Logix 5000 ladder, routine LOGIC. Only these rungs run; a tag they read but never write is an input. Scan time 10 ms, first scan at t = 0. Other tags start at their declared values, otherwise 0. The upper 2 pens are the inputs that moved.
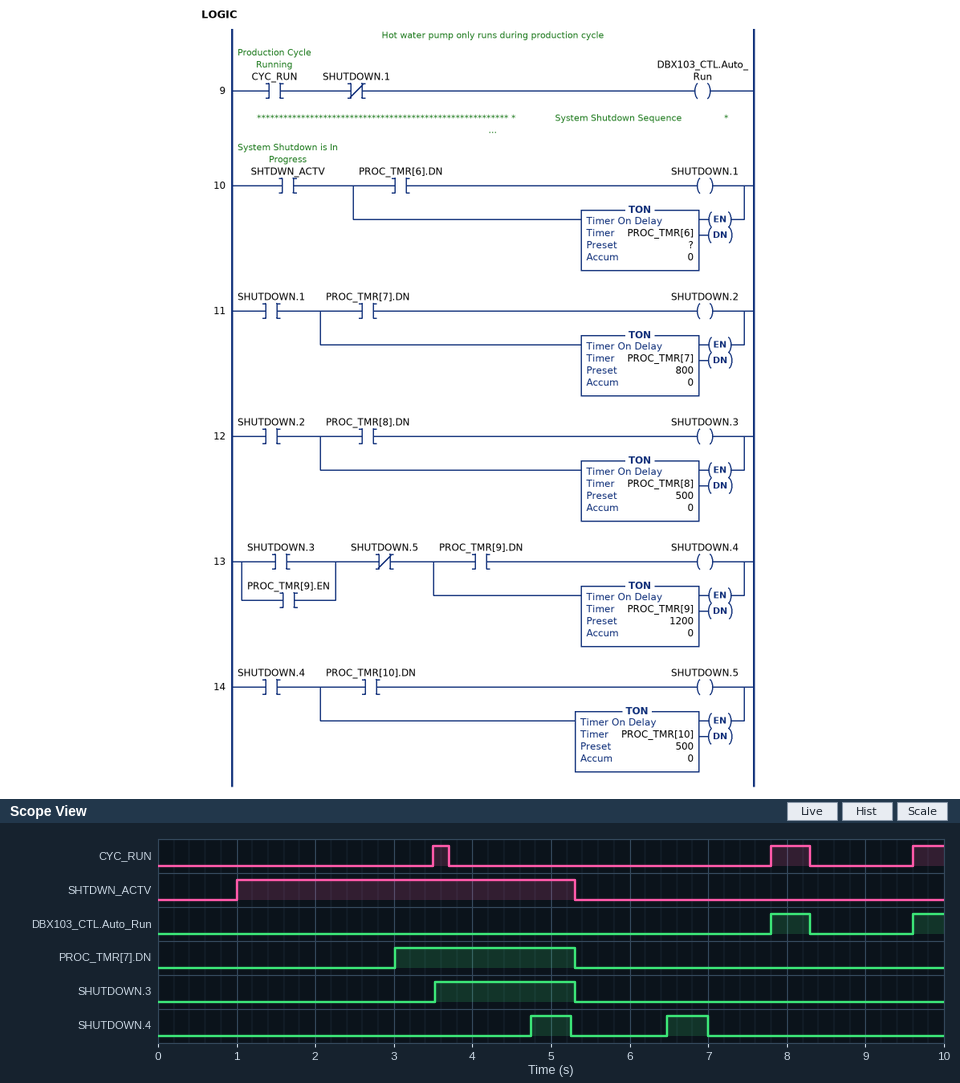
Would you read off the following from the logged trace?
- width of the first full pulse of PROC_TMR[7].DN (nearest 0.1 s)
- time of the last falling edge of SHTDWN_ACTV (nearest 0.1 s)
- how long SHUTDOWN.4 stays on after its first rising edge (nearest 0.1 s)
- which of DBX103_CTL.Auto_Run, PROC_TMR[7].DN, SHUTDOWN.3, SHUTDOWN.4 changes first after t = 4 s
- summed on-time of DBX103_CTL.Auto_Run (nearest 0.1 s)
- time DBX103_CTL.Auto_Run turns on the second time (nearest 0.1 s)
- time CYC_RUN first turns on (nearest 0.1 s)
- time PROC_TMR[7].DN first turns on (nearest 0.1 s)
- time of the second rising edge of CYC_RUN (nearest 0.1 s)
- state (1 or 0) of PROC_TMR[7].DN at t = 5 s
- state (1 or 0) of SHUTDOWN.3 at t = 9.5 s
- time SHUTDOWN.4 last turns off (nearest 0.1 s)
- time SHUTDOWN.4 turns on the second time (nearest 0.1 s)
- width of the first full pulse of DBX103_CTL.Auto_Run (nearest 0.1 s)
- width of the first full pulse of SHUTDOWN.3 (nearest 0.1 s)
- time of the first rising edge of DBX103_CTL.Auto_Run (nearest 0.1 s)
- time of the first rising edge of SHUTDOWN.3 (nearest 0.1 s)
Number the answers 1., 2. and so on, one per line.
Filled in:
1. 2.3 s
2. 5.3 s
3. 0.5 s
4. SHUTDOWN.4
5. 0.9 s
6. 9.6 s
7. 3.5 s
8. 3.0 s
9. 7.8 s
10. 1
11. 0
12. 7.0 s
13. 6.5 s
14. 0.5 s
15. 1.8 s
16. 7.8 s
17. 3.5 s
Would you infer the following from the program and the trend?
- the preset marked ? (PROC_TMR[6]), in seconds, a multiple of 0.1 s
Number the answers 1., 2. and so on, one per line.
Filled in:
1. 1.2 s
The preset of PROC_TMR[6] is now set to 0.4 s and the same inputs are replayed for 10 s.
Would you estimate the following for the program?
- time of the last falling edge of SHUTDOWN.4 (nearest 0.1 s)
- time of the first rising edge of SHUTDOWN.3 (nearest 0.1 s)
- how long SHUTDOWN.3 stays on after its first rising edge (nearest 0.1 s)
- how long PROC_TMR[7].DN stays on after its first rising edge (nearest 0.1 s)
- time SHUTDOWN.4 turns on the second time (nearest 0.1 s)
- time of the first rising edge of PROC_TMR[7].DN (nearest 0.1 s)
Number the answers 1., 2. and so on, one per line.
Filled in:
1. 6.2 s
2. 2.7 s
3. 2.6 s
4. 3.1 s
5. 5.7 s
6. 2.2 s
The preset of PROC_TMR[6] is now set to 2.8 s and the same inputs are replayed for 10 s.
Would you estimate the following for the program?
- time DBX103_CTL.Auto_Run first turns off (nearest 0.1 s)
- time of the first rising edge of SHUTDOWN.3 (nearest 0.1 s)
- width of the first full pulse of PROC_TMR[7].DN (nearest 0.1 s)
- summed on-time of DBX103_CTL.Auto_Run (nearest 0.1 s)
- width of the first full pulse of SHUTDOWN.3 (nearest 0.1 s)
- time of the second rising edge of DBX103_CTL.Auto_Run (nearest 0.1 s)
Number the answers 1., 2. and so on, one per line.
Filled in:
1. 3.7 s
2. 5.1 s
3. 0.7 s
4. 1.1 s
5. 0.2 s
6. 7.8 s
